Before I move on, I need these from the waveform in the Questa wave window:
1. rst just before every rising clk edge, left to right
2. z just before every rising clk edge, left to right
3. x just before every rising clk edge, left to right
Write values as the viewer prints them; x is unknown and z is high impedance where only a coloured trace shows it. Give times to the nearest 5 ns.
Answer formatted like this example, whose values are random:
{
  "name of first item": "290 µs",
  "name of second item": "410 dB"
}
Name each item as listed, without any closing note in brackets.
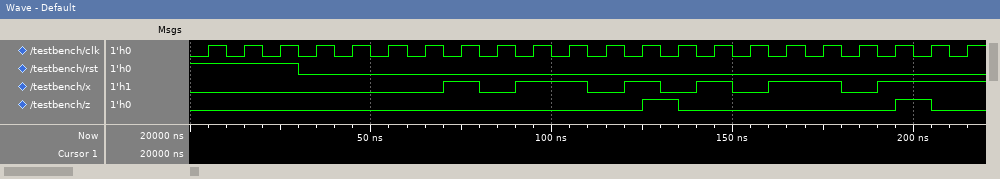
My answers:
{
  "rst just before every rising clk edge, left to right": "1 1 1 0 0 0 0 0 0 0 0 0 0 0 0 0 0 0 0 0 0 0",
  "z just before every rising clk edge, left to right": "0 0 0 0 0 0 0 0 0 0 0 0 0 1 0 0 0 0 0 0 1 0",
  "x just before every rising clk edge, left to right": "0 0 0 0 0 0 0 1 0 1 1 0 1 0 1 0 1 1 0 1 1 1"
}
